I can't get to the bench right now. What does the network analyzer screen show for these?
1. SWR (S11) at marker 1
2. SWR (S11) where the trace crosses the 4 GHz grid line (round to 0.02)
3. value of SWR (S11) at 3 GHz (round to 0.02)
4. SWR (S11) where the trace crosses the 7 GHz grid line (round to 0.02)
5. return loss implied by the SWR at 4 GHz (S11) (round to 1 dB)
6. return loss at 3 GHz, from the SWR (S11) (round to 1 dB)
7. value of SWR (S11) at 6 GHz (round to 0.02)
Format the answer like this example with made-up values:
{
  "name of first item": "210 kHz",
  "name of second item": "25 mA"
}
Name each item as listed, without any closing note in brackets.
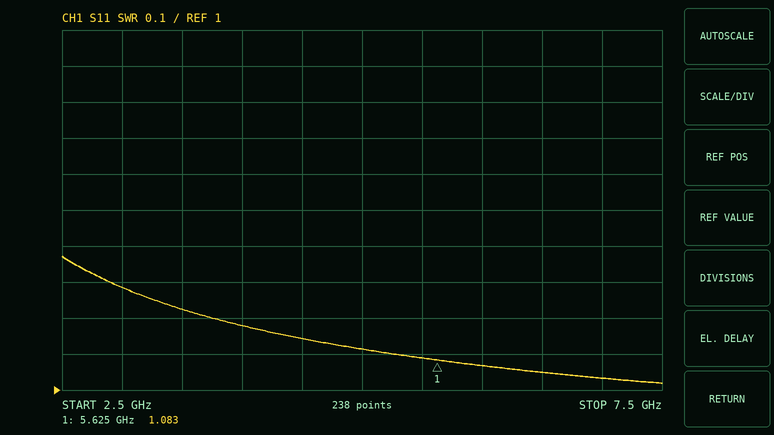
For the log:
{
  "SWR (S11) at marker 1": "1.083",
  "SWR (S11) where the trace crosses the 4 GHz grid line": "1.18",
  "value of SWR (S11) at 3 GHz": "1.28",
  "SWR (S11) where the trace crosses the 7 GHz grid line": "1.04",
  "return loss implied by the SWR at 4 GHz (S11)": "22 dB",
  "return loss at 3 GHz, from the SWR (S11)": "18 dB",
  "value of SWR (S11) at 6 GHz": "1.06"
}
